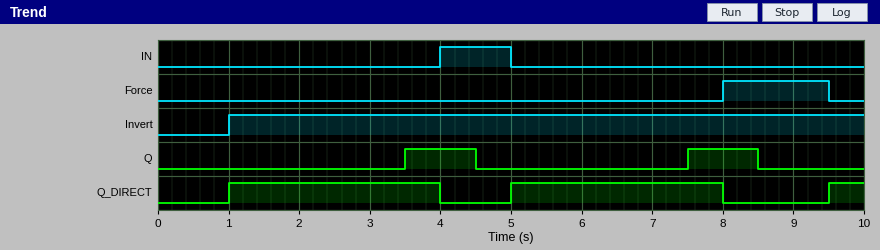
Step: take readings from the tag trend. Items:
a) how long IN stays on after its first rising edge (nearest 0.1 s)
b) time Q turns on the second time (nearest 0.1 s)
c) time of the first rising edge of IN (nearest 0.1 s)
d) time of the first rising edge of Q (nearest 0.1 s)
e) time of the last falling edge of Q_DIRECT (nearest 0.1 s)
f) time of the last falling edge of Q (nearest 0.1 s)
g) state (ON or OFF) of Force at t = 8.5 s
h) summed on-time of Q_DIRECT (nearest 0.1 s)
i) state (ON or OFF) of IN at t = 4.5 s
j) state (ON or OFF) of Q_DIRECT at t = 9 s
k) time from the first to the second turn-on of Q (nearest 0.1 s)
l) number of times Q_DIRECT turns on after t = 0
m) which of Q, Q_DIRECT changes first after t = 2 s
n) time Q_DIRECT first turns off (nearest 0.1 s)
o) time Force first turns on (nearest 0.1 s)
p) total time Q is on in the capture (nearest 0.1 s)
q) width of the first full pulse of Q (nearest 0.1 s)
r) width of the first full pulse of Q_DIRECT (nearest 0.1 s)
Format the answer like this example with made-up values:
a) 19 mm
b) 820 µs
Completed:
a) 1.0 s
b) 7.5 s
c) 4.0 s
d) 3.5 s
e) 8.0 s
f) 8.5 s
g) ON
h) 6.5 s
i) ON
j) OFF
k) 4.0 s
l) 3
m) Q
n) 4.0 s
o) 8.0 s
p) 2.0 s
q) 1.0 s
r) 3.0 s
